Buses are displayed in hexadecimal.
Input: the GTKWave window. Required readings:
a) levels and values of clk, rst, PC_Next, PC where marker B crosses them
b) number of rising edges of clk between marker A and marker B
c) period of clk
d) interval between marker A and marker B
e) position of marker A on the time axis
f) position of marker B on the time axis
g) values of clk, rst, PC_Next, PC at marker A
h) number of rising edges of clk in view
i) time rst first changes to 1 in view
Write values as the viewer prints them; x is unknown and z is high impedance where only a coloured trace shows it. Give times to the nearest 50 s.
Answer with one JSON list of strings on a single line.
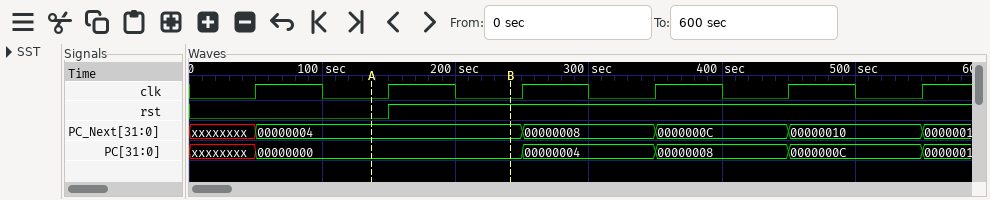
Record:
["clk=0, rst=1, PC_Next=00000004, PC=00000000", "1", "100 s", "100 s", "150 s", "250 s", "clk=0, rst=0, PC_Next=00000004, PC=00000000", "6", "150 s"]
